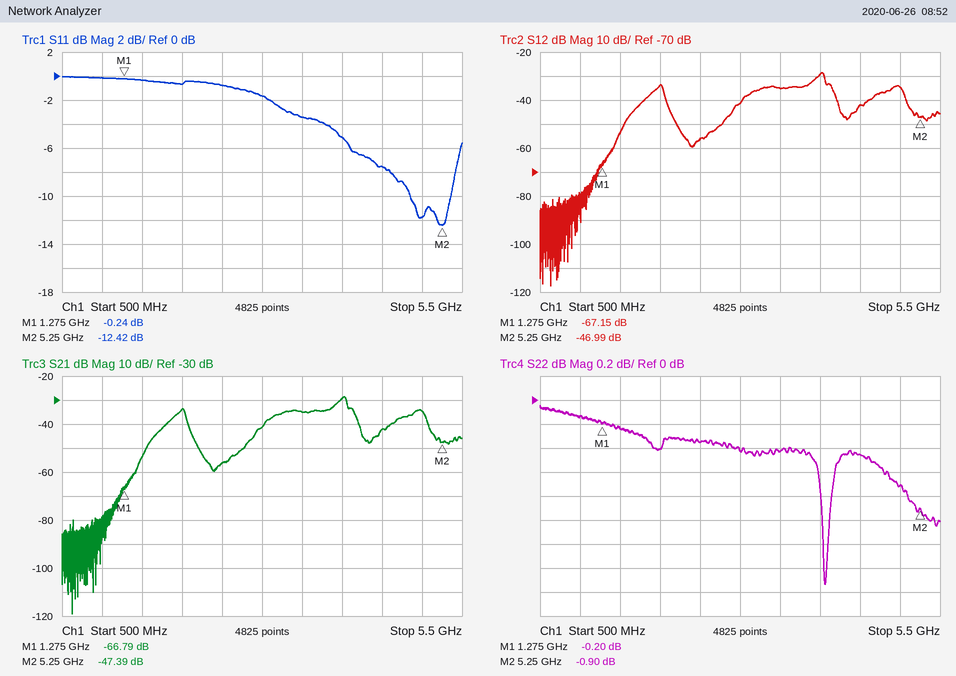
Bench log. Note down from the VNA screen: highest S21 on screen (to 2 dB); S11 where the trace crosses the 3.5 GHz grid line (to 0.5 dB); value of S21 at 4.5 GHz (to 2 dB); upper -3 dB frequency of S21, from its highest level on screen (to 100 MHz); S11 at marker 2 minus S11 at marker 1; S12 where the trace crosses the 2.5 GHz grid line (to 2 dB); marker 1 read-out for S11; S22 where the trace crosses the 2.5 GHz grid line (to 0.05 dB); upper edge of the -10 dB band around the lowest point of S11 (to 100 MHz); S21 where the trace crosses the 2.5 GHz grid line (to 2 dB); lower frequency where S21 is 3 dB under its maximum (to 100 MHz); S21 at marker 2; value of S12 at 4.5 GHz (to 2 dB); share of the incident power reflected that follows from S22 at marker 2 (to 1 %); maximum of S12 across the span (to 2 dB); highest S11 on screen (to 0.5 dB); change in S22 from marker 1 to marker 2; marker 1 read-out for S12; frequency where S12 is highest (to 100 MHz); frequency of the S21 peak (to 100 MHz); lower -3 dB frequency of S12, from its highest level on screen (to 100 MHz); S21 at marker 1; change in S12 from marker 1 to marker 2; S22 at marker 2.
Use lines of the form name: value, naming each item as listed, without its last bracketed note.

highest S21 on screen: -28 dB
S11 where the trace crosses the 3.5 GHz grid line: -3.5 dB
value of S21 at 4.5 GHz: -42 dB
upper -3 dB frequency of S21, from its highest level on screen: 4.1 GHz
S11 at marker 2 minus S11 at marker 1: -12.18 dB
S12 where the trace crosses the 2.5 GHz grid line: -56 dB
marker 1 read-out for S11: -0.24 dB
S22 where the trace crosses the 2.5 GHz grid line: -0.35 dB
upper edge of the -10 dB band around the lowest point of S11: 5.4 GHz
S21 where the trace crosses the 2.5 GHz grid line: -56 dB
lower frequency where S21 is 3 dB under its maximum: 3.9 GHz
S21 at marker 2: -47.39 dB
value of S12 at 4.5 GHz: -42 dB
share of the incident power reflected that follows from S22 at marker 2: 81 %
maximum of S12 across the span: -28 dB
highest S11 on screen: 0.0 dB
change in S22 from marker 1 to marker 2: -0.70 dB
marker 1 read-out for S12: -67.15 dB
frequency where S12 is highest: 4.0 GHz
frequency of the S21 peak: 4.0 GHz
lower -3 dB frequency of S12, from its highest level on screen: 3.9 GHz
S21 at marker 1: -66.79 dB
change in S12 from marker 1 to marker 2: 20.16 dB
S22 at marker 2: -0.90 dB
